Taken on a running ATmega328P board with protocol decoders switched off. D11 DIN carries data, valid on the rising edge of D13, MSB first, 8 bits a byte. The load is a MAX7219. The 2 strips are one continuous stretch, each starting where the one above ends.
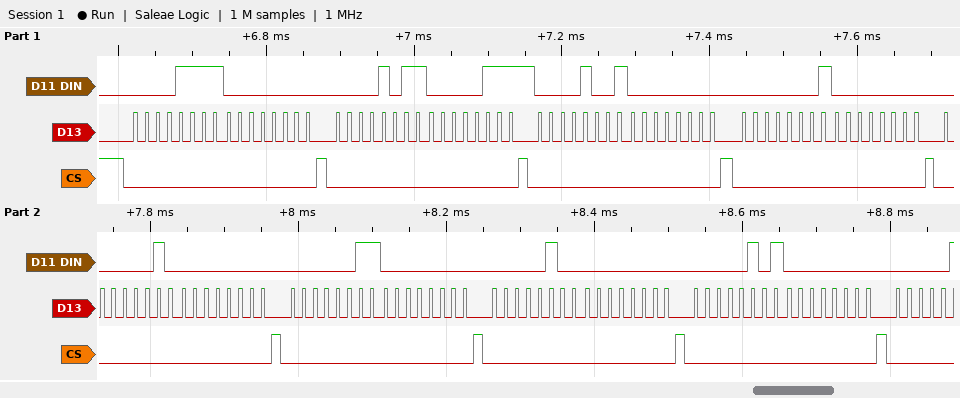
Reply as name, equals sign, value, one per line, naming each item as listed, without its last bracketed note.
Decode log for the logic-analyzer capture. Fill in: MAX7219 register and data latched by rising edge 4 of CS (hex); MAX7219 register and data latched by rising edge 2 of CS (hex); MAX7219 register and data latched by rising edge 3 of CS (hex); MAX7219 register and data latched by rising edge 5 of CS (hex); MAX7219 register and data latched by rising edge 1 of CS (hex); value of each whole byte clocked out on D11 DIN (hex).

MAX7219 register and data latched by rising edge 4 of CS = register 0x1, data 0x00
MAX7219 register and data latched by rising edge 2 of CS = register 0xB, data 0x07
MAX7219 register and data latched by rising edge 3 of CS = register 0x9, data 0x00
MAX7219 register and data latched by rising edge 5 of CS = register 0x2, data 0x00
MAX7219 register and data latched by rising edge 1 of CS = register 0xF, data 0x00
value of each whole byte clocked out on D11 DIN = 0x0F 0x00 0x0B 0x07 0x09 0x00 0x01 0x00 0x02 0x00 0x03 0x00 0x04 0x00 0x05 0x00
